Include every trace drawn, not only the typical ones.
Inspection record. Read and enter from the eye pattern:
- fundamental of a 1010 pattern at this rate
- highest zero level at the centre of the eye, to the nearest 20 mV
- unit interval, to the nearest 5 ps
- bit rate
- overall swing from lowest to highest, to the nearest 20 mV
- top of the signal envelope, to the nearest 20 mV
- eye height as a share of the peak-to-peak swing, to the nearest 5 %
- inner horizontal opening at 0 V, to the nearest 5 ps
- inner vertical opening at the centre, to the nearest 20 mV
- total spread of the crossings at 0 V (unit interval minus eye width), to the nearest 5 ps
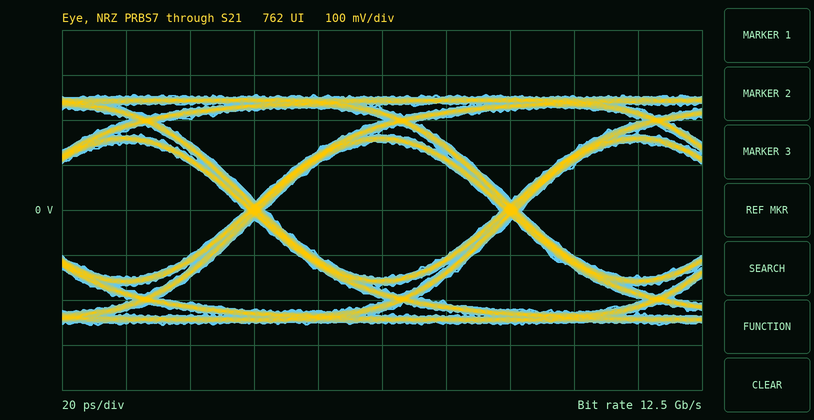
6.25 GHz
-160 mV
80 ps
12.5 Gb/s
520 mV
260 mV
60 %
75 ps
300 mV
5 ps
